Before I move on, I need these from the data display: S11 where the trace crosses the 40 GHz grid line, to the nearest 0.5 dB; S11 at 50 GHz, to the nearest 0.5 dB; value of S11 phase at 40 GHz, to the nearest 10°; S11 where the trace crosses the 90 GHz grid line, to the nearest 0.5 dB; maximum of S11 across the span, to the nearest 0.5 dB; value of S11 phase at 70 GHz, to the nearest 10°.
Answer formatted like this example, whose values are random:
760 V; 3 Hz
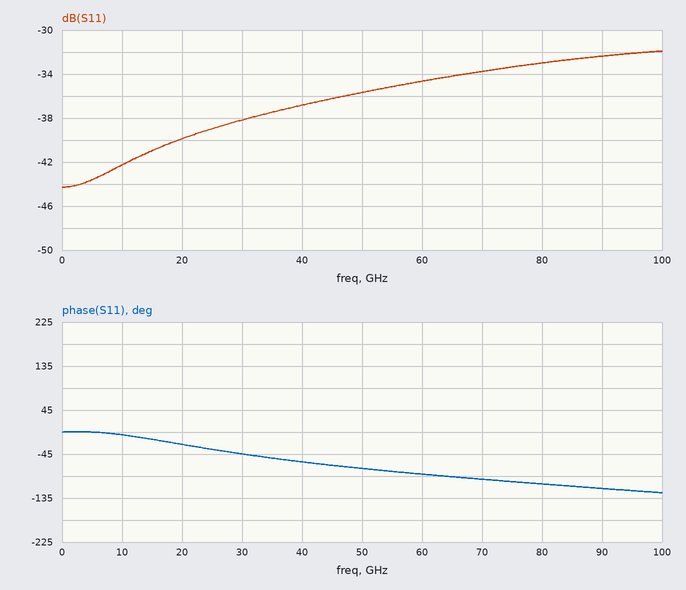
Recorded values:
-37.0 dB; -35.5 dB; -60°; -32.5 dB; -32.0 dB; -100°
